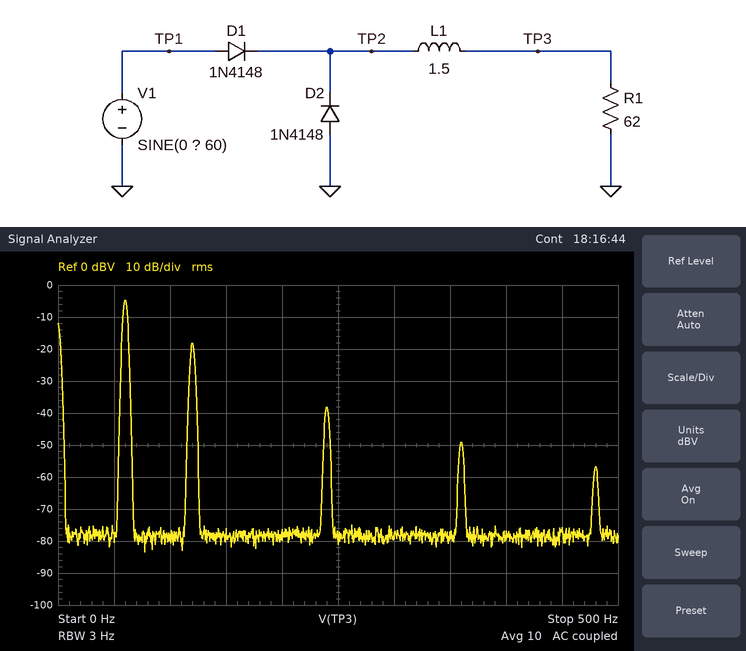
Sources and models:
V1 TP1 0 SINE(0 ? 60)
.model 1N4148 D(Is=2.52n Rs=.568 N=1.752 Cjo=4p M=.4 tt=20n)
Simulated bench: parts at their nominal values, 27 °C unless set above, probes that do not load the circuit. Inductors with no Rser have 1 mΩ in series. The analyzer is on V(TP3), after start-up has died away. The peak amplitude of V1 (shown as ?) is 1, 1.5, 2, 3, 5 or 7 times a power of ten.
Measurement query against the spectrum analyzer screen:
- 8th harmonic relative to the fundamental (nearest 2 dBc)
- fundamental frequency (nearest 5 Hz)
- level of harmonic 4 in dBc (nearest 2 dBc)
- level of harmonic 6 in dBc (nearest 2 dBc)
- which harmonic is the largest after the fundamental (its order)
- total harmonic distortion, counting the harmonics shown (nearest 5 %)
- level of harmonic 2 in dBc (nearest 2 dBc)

-52 dBc
60 Hz
-34 dBc
-44 dBc
2
20 %
-14 dBc
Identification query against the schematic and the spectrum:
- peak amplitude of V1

15 V
